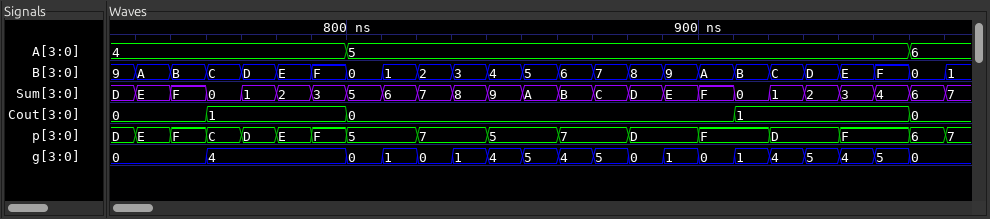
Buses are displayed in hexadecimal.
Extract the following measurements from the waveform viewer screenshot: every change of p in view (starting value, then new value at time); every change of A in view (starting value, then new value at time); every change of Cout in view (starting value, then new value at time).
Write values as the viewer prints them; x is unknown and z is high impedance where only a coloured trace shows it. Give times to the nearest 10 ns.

D, E at 740 ns, F at 750 ns, C at 760 ns, D at 770 ns, E at 780 ns, F at 790 ns, 5 at 800 ns, 7 at 820 ns, 5 at 840 ns, 7 at 860 ns, D at 880 ns, F at 900 ns, D at 920 ns, F at 940 ns, 6 at 960 ns, 7 at 970 ns
4, 5 at 800 ns, 6 at 960 ns
0, 1 at 760 ns, 0 at 800 ns, 1 at 910 ns, 0 at 960 ns
